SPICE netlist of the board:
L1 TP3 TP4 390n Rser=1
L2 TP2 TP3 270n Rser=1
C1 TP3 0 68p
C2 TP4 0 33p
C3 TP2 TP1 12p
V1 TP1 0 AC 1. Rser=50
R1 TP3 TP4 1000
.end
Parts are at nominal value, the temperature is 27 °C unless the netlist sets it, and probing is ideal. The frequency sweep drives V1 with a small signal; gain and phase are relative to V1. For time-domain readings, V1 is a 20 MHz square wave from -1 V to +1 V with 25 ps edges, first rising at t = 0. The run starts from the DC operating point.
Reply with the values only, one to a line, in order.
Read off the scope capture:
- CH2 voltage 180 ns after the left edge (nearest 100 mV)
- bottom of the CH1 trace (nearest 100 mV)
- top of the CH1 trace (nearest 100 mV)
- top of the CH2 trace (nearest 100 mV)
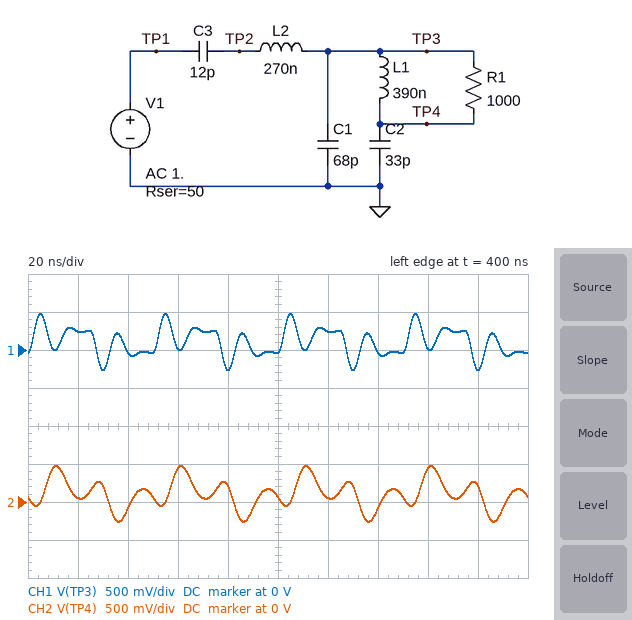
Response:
200 mV
-300 mV
500 mV
500 mV
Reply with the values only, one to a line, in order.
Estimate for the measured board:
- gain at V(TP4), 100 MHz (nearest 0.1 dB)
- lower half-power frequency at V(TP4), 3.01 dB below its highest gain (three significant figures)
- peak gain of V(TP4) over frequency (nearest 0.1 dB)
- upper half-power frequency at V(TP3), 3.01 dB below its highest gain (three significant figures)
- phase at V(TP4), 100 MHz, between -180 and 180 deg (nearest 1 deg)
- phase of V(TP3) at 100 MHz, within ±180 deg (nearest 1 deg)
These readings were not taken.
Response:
-18.0 dB
48.3 MHz
-0.1 dB
108 MHz
98 deg
-99 deg
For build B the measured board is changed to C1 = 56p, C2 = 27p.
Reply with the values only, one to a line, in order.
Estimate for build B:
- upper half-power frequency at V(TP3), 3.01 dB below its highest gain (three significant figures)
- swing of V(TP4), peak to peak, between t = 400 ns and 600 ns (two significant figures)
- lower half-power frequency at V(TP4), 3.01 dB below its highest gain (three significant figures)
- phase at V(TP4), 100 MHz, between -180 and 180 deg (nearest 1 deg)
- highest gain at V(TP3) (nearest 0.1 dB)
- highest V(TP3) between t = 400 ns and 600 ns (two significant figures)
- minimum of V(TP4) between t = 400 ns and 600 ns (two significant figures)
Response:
110 MHz
1.3 V
52.4 MHz
108 deg
-3.7 dB
560 mV
-500 mV
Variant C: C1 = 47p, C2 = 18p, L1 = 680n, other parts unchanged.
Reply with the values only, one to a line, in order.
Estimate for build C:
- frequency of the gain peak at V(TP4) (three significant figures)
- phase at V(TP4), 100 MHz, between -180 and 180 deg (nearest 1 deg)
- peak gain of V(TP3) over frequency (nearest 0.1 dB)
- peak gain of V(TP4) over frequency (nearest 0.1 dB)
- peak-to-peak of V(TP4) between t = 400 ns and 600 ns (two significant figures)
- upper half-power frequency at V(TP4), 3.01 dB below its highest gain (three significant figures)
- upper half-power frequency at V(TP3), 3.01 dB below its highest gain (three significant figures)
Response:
51.2 MHz
123 deg
-3.0 dB
-0.9 dB
960 mV
57.5 MHz
112 MHz
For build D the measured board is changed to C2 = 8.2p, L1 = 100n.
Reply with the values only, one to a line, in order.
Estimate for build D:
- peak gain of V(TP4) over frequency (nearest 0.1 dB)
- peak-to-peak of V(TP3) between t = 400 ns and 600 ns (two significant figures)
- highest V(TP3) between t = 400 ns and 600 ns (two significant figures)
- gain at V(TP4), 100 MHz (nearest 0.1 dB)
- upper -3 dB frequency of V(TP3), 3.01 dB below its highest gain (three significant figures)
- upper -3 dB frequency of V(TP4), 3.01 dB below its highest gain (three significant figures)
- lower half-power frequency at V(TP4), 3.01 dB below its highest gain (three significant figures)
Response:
-4.7 dB
580 mV
430 mV
-5.3 dB
106 MHz
110 MHz
79.1 MHz
